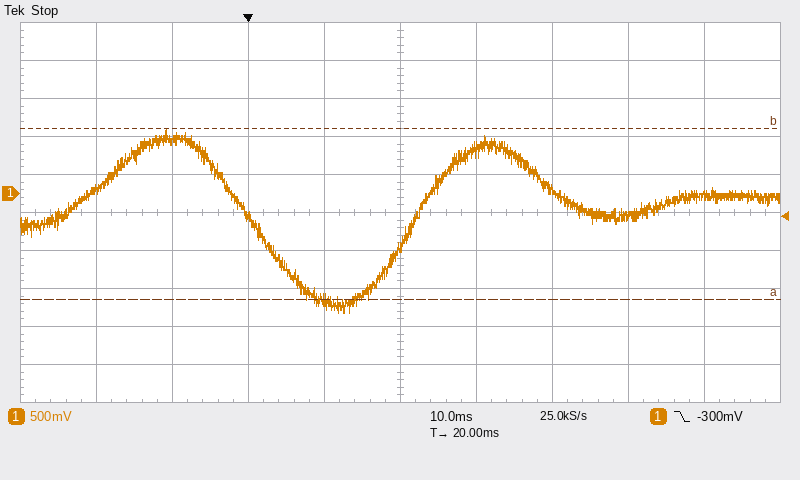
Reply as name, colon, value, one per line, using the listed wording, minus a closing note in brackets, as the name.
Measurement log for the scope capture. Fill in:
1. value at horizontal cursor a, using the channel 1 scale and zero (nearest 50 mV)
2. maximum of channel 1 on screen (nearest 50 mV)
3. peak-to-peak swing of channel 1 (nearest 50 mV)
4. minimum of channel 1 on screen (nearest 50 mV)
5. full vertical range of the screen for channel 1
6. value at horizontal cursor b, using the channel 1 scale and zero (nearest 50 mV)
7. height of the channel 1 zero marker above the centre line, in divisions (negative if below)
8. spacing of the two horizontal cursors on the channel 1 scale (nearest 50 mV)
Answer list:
value at horizontal cursor a, using the channel 1 scale and zero: -1.40 V
maximum of channel 1 on screen: 850 mV
peak-to-peak swing of channel 1: 2.40 V
minimum of channel 1 on screen: -1.55 V
full vertical range of the screen for channel 1: 5 V
value at horizontal cursor b, using the channel 1 scale and zero: 850 mV
height of the channel 1 zero marker above the centre line, in divisions: +0.5 div
spacing of the two horizontal cursors on the channel 1 scale: 2.25 V
